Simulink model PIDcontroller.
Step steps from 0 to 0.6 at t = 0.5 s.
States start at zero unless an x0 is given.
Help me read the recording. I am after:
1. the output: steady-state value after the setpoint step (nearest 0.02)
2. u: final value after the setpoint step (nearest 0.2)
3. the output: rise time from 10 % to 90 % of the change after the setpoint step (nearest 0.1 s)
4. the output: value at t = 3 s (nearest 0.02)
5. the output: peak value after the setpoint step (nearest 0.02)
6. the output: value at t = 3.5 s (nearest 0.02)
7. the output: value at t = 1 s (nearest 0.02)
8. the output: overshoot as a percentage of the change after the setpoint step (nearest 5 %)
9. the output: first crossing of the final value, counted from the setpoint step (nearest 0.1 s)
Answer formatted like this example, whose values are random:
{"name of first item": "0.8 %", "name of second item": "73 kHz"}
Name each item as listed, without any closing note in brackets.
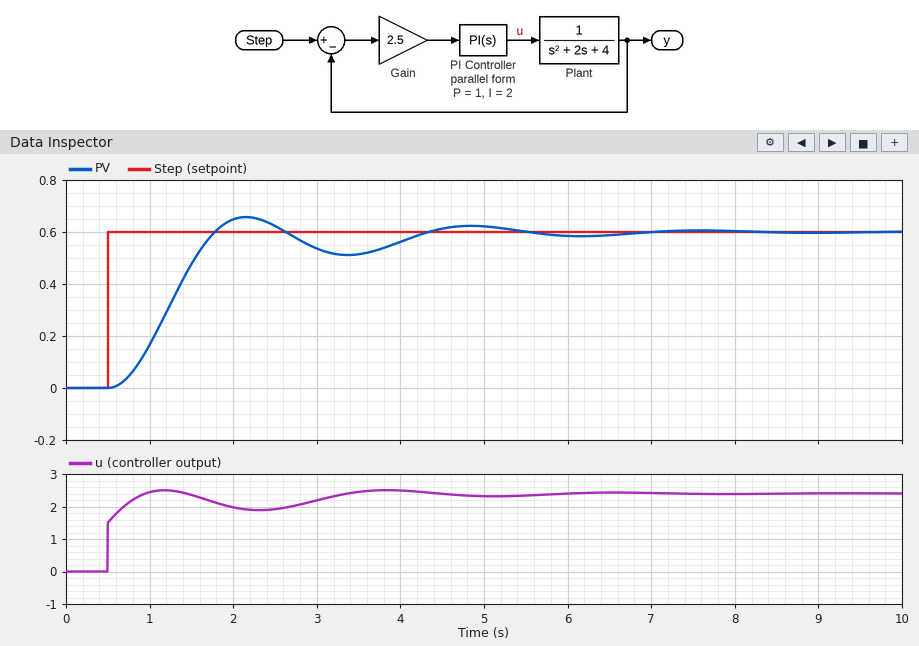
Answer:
{"the output: steady-state value after the setpoint step": "0.60", "u: final value after the setpoint step": "2.4", "the output: rise time from 10 % to 90 % of the change after the setpoint step": "0.8 s", "the output: value at t = 3 s": "0.54", "the output: peak value after the setpoint step": "0.66", "the output: value at t = 3.5 s": "0.52", "the output: value at t = 1 s": "0.16", "the output: overshoot as a percentage of the change after the setpoint step": "10 %", "the output: first crossing of the final value, counted from the setpoint step": "1.3 s"}
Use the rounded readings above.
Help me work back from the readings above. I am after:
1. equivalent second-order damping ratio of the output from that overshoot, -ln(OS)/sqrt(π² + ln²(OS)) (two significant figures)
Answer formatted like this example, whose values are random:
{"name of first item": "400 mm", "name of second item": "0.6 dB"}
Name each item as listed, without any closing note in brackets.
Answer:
{"equivalent second-order damping ratio of the output from that overshoot, -ln(OS)/sqrt(π² + ln²(OS))": "0.59"}
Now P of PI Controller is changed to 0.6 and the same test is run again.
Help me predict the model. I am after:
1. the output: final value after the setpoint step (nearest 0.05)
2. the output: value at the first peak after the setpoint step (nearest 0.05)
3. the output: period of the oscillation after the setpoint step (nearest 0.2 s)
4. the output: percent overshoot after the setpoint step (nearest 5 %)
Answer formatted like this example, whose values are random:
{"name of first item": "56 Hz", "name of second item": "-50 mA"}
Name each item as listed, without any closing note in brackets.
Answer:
{"the output: final value after the setpoint step": "0.60", "the output: value at the first peak after the setpoint step": "0.70", "the output: period of the oscillation after the setpoint step": "3.0 s", "the output: percent overshoot after the setpoint step": "15 %"}
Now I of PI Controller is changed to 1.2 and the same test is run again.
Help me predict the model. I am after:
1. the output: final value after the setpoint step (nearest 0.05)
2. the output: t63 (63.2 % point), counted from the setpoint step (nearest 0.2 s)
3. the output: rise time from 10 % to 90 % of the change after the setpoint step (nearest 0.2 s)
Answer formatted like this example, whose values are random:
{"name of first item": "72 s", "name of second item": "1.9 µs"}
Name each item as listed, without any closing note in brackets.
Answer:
{"the output: final value after the setpoint step": "0.60", "the output: t63 (63.2 % point), counted from the setpoint step": "1.0 s", "the output: rise time from 10 % to 90 % of the change after the setpoint step": "3.4 s"}
